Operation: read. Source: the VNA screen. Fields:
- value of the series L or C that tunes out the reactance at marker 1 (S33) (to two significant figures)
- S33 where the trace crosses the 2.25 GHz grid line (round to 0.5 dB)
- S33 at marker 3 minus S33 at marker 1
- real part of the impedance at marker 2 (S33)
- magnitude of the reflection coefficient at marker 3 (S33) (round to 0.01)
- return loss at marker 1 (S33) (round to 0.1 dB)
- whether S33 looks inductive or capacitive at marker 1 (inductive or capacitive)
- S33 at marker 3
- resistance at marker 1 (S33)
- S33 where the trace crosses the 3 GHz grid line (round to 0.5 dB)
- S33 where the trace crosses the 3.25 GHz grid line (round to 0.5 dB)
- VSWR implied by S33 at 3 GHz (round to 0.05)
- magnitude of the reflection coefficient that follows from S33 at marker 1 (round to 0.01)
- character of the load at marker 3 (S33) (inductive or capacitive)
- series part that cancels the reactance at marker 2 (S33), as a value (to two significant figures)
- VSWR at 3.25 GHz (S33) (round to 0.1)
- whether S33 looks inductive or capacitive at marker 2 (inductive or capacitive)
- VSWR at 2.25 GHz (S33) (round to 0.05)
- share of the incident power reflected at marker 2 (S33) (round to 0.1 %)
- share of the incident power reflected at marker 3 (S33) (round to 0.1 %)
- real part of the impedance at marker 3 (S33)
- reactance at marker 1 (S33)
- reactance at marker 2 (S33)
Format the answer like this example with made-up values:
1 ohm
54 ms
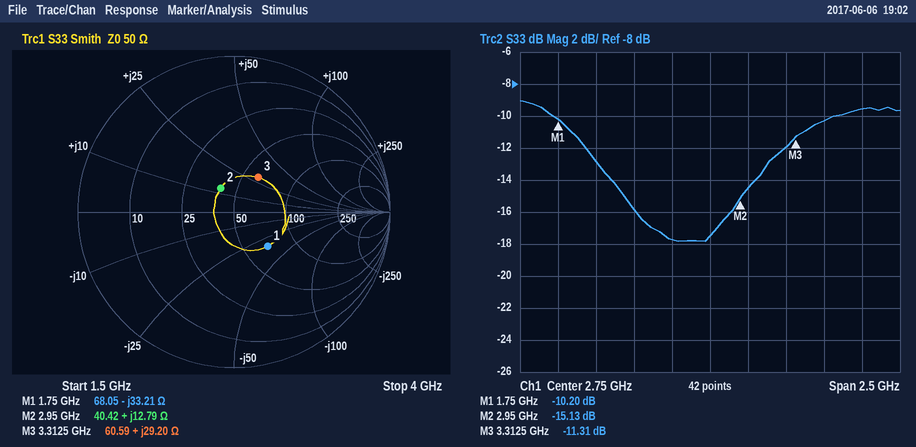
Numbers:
3.0 nH
-16.0 dB
-1.11 dB
40.42 Ω
0.27
10.2 dB
capacitive
-11.31 dB
68.05 Ω
-14.5 dB
-12.0 dB
1.45
0.31
inductive
4.2 pF
1.7
inductive
1.40
3.1 %
7.4 %
60.59 Ω
-33.21 Ω
+12.79 Ω
